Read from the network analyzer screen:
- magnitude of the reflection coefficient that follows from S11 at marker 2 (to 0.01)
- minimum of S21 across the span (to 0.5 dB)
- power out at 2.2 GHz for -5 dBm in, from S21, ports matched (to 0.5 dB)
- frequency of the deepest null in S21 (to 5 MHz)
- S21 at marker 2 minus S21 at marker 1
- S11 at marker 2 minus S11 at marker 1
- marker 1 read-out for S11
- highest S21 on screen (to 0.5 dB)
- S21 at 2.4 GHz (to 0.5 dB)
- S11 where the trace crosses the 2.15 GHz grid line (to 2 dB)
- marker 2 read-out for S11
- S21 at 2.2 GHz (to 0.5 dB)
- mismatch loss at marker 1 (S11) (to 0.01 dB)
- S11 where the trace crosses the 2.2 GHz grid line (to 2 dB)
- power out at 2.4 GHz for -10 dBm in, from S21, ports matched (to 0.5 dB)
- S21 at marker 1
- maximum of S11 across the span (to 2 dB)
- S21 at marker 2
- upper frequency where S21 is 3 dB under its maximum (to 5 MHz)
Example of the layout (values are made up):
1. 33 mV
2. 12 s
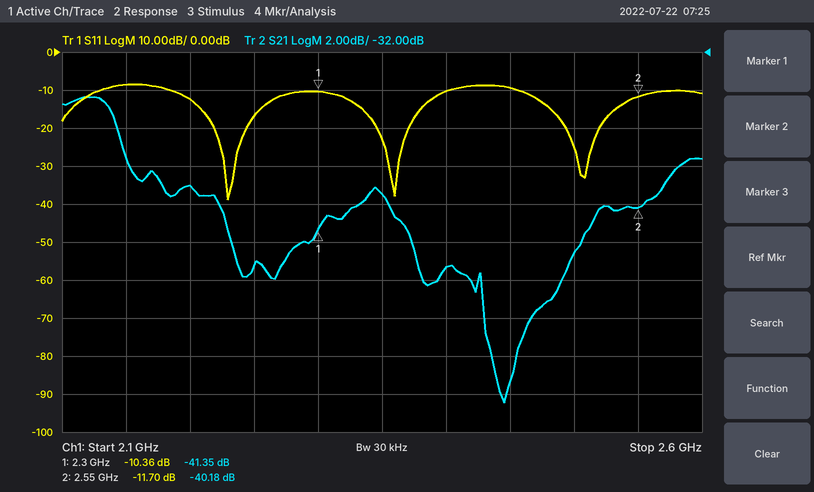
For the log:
1. 0.26
2. -50.5 dB
3. -44.0 dBm
4. 2.445 GHz
5. 1.17 dB
6. -1.34 dB
7. -10.36 dB
8. -34.5 dB
9. -43.5 dB
10. -8 dB
11. -11.70 dB
12. -39.0 dB
13. 0.42 dB
14. -12 dB
15. -53.5 dBm
16. -41.35 dB
17. -8 dB
18. -40.18 dB
19. 2.150 GHz
